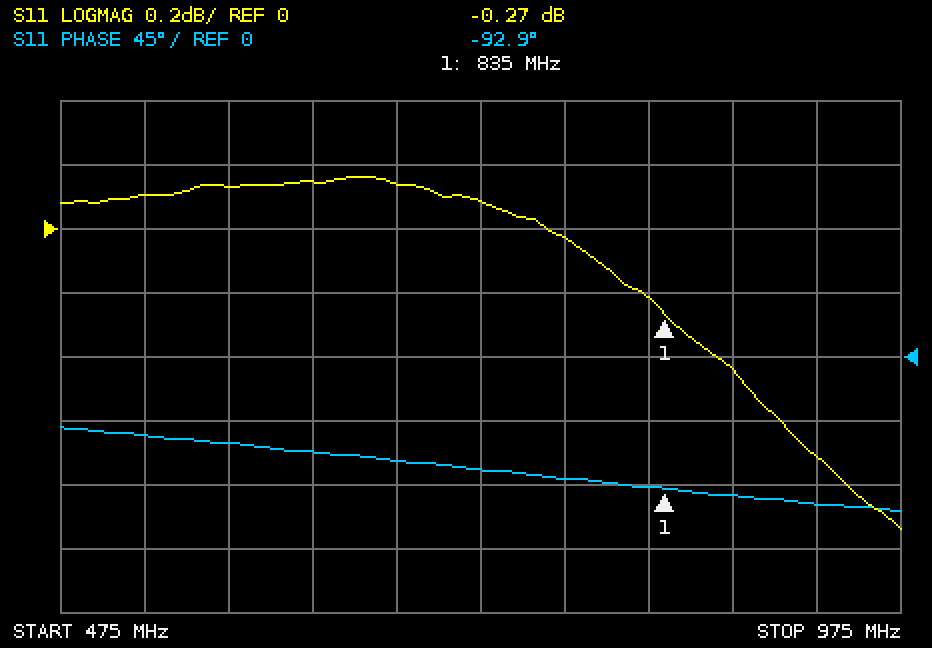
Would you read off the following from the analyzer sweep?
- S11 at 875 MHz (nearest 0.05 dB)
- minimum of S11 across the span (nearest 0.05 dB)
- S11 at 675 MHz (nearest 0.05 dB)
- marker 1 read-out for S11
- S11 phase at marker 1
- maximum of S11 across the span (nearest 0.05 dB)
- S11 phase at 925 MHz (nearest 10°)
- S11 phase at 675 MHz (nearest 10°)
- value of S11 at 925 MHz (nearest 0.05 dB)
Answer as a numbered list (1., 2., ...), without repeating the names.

1. -0.45 dB
2. -0.95 dB
3. 0.15 dB
4. -0.27 dB
5. -92.9°
6. 0.15 dB
7. -100°
8. -70°
9. -0.70 dB
